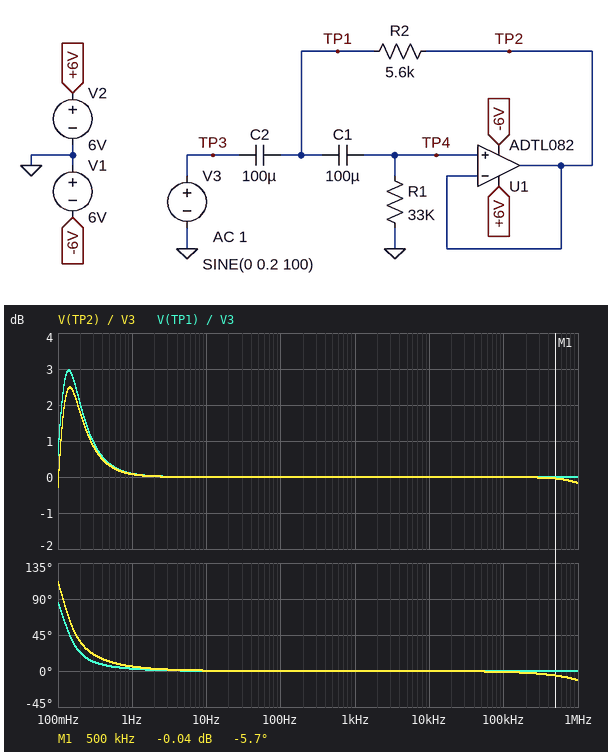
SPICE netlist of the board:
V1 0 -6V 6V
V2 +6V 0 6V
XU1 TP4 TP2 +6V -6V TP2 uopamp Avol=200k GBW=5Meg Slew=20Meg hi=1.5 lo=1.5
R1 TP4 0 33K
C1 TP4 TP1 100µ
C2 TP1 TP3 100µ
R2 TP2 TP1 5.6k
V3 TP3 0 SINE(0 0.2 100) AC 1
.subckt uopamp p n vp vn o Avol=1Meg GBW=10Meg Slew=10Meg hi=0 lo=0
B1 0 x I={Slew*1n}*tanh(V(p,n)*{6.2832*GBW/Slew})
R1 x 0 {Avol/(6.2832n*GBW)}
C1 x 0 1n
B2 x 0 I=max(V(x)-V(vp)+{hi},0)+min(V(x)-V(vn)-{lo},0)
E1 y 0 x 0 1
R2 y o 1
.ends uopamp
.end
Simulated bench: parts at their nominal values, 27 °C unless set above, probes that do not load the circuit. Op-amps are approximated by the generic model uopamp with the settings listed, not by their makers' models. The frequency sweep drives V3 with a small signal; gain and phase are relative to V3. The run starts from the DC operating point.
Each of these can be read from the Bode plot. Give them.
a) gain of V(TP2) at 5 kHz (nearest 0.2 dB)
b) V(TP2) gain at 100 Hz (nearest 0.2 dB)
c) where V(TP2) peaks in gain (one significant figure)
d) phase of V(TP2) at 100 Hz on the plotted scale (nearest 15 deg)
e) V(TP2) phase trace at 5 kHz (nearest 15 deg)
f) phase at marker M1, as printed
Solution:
0 dB
0 dB
100 mHz
0 deg
0 deg
-5.7 deg
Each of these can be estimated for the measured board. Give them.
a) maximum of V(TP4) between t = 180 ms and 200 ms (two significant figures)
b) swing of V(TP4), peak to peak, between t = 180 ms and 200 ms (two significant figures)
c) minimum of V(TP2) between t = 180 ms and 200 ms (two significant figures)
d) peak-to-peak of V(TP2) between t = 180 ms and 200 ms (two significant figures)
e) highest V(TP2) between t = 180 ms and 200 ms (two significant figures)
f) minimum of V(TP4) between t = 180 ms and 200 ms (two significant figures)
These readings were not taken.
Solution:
200 mV
400 mV
-200 mV
400 mV
200 mV
-200 mV
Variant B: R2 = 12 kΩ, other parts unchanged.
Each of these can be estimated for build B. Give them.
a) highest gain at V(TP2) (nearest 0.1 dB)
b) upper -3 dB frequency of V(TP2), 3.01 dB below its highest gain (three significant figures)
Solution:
0.3 dB
4.61 MHz
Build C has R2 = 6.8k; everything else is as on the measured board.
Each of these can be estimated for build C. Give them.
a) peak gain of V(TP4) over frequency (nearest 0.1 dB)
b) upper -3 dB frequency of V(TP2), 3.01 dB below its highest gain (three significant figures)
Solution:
1.8 dB
2.78 MHz
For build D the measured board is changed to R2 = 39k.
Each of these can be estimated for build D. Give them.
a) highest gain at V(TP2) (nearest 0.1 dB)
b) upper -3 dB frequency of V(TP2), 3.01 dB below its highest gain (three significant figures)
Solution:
0 dB
5.00 MHz
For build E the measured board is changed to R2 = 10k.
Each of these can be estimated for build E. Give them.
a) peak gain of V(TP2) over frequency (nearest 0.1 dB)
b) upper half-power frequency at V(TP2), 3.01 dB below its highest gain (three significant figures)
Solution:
0.7 dB
4.15 MHz
